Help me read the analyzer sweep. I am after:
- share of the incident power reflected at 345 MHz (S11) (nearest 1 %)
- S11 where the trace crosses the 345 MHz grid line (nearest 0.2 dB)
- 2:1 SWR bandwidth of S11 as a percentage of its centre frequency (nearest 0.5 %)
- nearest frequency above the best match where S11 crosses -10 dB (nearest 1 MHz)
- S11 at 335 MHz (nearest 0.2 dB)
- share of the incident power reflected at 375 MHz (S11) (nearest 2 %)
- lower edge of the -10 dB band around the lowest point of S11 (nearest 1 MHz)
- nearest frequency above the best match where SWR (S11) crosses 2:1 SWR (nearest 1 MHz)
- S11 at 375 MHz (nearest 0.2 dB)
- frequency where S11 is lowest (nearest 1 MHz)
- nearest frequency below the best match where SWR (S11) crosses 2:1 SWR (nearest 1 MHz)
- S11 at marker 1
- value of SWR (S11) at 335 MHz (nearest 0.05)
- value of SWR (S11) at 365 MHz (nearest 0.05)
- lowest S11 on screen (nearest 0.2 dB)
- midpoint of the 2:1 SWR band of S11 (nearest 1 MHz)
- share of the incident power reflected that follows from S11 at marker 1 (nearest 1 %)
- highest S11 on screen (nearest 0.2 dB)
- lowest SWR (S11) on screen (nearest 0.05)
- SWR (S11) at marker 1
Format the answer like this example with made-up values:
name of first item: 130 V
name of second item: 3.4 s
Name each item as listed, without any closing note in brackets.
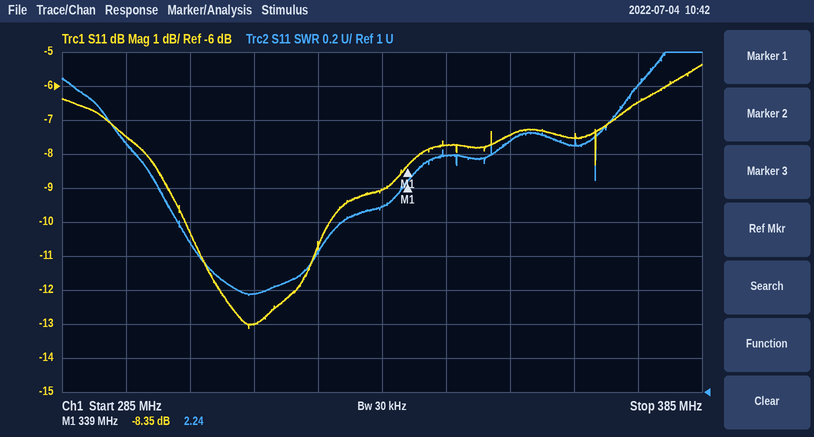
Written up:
share of the incident power reflected at 345 MHz (S11): 17 %
S11 where the trace crosses the 345 MHz grid line: -7.8 dB
2:1 SWR bandwidth of S11 as a percentage of its centre frequency: 8.0 %
nearest frequency above the best match where S11 crosses -10 dB: 327 MHz
S11 at 335 MHz: -9.0 dB
share of the incident power reflected at 375 MHz (S11): 22 %
lower edge of the -10 dB band around the lowest point of S11: 304 MHz
nearest frequency above the best match where SWR (S11) crosses 2:1 SWR: 329 MHz
S11 at 375 MHz: -6.4 dB
frequency where S11 is lowest: 314 MHz
nearest frequency below the best match where SWR (S11) crosses 2:1 SWR: 303 MHz
S11 at marker 1: -8.35 dB
value of SWR (S11) at 335 MHz: 2.10
value of SWR (S11) at 365 MHz: 2.45
lowest S11 on screen: -13.2 dB
midpoint of the 2:1 SWR band of S11: 316 MHz
share of the incident power reflected that follows from S11 at marker 1: 15 %
highest S11 on screen: -5.4 dB
lowest SWR (S11) on screen: 1.55
SWR (S11) at marker 1: 2.24
